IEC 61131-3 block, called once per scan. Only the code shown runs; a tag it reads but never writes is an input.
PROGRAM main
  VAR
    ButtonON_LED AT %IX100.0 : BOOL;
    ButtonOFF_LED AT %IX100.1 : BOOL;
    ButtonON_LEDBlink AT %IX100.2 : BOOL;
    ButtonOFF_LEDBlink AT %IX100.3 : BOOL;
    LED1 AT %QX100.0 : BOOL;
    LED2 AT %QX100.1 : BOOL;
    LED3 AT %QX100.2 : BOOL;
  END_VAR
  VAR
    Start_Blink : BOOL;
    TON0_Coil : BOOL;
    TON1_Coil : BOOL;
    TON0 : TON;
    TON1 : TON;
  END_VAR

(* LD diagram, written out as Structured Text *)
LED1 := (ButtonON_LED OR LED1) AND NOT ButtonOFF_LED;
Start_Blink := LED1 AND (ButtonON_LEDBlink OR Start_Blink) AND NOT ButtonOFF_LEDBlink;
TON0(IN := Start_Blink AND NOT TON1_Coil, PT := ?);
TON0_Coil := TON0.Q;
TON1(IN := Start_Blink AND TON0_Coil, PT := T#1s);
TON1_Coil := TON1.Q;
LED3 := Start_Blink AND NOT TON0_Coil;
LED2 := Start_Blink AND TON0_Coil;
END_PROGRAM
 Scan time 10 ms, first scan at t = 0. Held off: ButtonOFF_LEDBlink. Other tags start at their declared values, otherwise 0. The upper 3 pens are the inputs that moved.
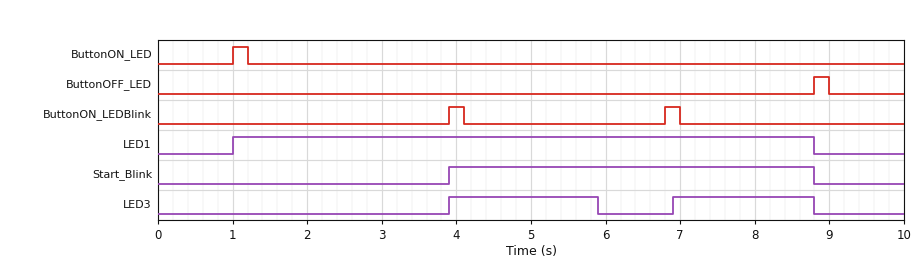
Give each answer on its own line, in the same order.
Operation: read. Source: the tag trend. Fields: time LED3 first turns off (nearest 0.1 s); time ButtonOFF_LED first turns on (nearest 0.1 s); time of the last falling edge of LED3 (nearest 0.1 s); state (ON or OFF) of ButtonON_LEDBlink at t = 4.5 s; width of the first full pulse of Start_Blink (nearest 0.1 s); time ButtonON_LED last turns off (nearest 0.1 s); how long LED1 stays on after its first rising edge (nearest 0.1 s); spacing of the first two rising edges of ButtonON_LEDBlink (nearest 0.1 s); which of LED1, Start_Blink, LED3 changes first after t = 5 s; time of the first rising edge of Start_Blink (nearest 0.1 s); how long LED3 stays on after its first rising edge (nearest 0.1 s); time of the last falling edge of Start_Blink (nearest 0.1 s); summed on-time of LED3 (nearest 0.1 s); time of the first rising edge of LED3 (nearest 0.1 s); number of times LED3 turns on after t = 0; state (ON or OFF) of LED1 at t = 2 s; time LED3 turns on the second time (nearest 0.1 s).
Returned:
5.9 s
8.8 s
8.8 s
OFF
4.9 s
1.2 s
7.8 s
2.9 s
LED3
3.9 s
2.0 s
8.8 s
3.9 s
3.9 s
2
ON
6.9 s
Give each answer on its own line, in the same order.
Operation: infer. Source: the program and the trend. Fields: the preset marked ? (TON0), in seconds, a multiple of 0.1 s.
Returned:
2.0 s
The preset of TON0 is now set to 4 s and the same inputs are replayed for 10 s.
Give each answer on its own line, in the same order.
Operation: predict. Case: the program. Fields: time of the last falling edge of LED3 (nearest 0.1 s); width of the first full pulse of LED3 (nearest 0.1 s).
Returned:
7.9 s
4.0 s
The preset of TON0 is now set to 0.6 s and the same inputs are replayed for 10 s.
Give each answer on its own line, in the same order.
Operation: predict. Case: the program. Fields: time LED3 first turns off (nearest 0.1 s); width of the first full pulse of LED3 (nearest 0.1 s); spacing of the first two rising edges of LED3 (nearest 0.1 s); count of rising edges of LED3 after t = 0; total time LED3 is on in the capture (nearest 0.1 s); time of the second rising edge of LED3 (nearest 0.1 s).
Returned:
4.5 s
0.6 s
1.6 s
4
1.9 s
5.5 s
